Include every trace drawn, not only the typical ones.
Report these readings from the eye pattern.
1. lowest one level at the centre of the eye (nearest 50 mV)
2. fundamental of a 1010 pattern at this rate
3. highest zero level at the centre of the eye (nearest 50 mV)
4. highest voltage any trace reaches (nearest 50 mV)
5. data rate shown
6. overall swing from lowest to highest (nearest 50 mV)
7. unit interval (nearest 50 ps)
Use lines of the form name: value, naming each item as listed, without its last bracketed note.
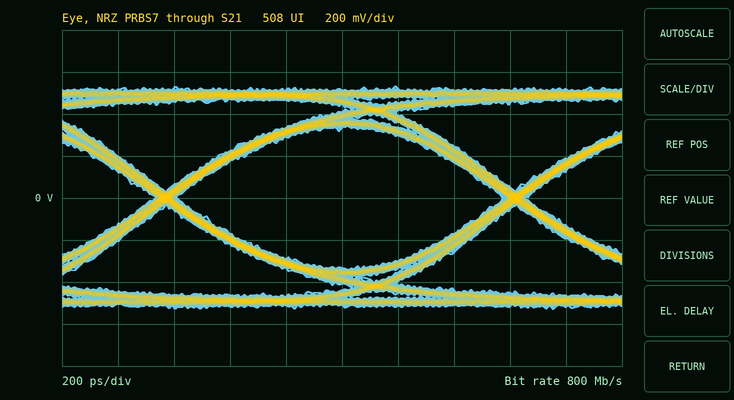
lowest one level at the centre of the eye: 350 mV
fundamental of a 1010 pattern at this rate: 400 MHz
highest zero level at the centre of the eye: -350 mV
highest voltage any trace reaches: 550 mV
data rate shown: 800 Mb/s
overall swing from lowest to highest: 1.05 V
unit interval: 1.25 ns
